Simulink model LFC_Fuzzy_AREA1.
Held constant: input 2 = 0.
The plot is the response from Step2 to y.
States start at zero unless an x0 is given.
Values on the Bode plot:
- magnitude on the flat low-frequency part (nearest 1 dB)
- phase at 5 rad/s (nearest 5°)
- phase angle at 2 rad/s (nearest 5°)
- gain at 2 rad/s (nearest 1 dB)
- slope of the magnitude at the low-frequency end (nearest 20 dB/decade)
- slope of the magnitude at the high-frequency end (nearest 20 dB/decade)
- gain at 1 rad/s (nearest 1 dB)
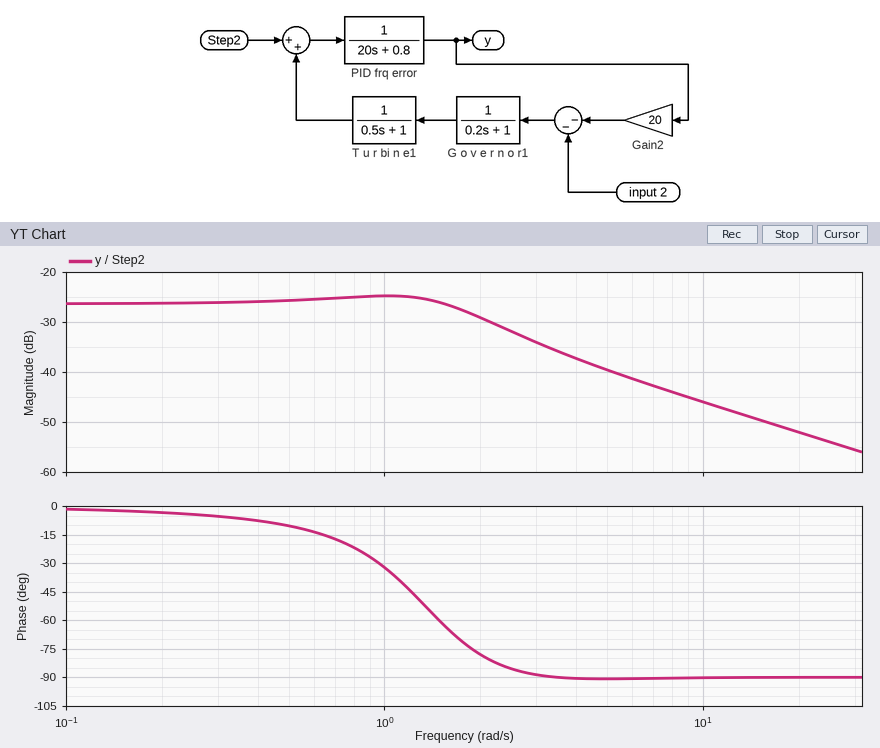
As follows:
-26 dB
-90°
-80°
-29 dB
0 dB/decade
-20 dB/decade
-25 dB
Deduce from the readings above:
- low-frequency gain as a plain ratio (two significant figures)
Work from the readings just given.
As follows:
0.050
